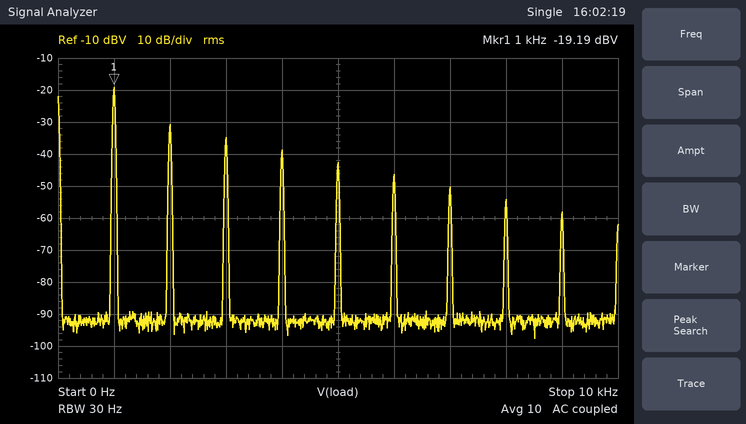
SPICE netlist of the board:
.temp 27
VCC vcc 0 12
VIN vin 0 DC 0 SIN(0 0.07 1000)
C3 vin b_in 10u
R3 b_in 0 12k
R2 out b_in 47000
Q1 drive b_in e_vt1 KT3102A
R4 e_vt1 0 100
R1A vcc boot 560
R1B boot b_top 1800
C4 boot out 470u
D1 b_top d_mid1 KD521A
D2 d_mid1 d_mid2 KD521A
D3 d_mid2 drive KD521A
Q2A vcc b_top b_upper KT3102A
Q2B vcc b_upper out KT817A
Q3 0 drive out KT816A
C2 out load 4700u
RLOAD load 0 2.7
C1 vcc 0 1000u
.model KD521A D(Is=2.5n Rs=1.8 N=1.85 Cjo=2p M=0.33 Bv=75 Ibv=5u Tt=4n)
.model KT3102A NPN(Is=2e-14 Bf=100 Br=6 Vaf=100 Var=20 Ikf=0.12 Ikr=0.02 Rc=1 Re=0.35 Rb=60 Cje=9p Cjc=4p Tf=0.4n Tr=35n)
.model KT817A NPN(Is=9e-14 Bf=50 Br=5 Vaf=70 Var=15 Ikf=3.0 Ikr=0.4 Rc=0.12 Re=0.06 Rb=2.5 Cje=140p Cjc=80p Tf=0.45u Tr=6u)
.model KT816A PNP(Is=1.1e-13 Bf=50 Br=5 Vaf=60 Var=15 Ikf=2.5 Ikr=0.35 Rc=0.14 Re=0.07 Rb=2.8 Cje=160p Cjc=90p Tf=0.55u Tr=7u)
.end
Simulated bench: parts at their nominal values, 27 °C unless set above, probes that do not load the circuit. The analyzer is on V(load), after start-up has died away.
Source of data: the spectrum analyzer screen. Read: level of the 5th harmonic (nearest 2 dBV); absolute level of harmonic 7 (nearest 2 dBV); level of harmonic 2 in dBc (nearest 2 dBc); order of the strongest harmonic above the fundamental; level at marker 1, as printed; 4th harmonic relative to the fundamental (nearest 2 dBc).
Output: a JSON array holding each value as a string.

["-42 dBV", "-50 dBV", "-12 dBc", "2", "-19.19 dBV", "-20 dBc"]
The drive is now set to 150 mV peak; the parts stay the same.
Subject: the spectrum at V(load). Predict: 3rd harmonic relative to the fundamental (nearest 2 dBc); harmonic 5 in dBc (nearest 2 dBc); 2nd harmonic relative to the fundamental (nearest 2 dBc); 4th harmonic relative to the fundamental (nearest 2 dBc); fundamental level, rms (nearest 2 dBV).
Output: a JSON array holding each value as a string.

["-8 dBc", "-14 dBc", "-6 dBc", "-10 dBc", "-10 dBV"]
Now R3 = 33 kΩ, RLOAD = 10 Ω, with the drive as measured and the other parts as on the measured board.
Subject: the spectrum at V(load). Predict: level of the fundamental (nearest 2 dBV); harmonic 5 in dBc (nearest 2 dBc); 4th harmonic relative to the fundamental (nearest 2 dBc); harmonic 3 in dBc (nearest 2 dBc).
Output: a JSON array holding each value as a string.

["-10 dBV", "-46 dBc", "-38 dBc", "-28 dBc"]
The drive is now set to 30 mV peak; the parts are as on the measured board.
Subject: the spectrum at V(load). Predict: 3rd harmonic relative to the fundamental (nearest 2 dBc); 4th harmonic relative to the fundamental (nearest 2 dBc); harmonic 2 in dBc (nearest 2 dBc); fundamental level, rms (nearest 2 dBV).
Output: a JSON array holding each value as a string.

["-36 dBc", "-48 dBc", "-24 dBc", "-28 dBV"]
